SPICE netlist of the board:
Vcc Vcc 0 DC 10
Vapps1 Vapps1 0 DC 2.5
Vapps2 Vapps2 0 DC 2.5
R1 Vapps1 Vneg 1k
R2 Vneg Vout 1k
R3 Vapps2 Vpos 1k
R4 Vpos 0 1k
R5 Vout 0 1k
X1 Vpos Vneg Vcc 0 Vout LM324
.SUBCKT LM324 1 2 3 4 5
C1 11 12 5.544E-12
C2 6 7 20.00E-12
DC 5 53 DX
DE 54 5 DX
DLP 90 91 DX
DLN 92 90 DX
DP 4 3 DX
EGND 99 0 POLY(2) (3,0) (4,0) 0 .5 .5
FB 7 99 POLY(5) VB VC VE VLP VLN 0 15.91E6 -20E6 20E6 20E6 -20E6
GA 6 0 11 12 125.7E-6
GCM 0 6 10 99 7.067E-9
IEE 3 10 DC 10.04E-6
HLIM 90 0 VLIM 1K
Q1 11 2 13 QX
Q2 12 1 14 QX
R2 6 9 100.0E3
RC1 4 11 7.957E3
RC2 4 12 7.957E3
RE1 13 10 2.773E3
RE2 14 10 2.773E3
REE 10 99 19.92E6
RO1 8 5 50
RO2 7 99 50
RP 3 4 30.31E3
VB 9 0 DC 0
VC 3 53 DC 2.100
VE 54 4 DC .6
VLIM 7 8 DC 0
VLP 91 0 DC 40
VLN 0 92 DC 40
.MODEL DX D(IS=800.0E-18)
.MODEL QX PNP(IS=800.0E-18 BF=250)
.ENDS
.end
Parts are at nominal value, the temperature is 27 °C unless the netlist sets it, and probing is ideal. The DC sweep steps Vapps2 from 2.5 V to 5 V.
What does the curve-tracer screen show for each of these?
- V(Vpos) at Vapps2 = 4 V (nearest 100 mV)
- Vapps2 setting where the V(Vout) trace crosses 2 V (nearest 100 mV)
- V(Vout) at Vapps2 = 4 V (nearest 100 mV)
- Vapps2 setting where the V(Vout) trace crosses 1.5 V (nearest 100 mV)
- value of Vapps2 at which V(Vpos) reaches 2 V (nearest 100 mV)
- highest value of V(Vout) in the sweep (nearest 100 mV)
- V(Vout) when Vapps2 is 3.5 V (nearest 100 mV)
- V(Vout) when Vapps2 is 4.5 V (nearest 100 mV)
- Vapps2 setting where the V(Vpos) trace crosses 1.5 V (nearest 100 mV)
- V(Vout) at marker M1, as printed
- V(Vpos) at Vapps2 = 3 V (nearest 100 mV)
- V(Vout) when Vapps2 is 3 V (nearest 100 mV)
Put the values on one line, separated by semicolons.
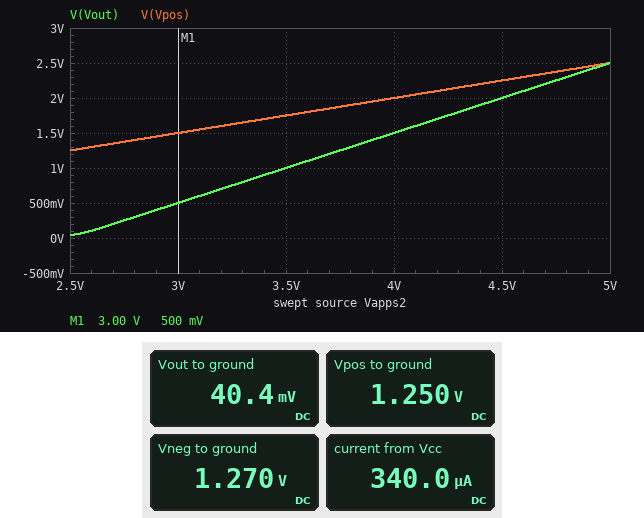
2.0 V; 4.5 V; 1.5 V; 4.0 V; 4.0 V; 2.5 V; 1.0 V; 2.0 V; 3.0 V; 500 mV; 1.5 V; 500 mV
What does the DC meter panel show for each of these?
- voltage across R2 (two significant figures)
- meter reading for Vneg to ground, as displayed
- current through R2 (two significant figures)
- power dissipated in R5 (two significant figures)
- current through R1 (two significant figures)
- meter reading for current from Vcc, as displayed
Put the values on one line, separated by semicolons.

1.2 V; 1.270 V; 1.2 mA; 1.6 µW; 1.2 mA; 340.0 µA
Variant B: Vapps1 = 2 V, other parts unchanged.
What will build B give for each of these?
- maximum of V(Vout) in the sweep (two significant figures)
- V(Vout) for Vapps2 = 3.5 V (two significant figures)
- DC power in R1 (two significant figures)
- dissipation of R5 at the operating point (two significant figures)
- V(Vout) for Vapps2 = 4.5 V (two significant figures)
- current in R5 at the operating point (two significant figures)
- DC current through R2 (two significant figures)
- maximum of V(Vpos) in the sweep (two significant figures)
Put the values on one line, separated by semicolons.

3.0 V; 1.5 V; 560 µW; 250 µW; 2.5 V; 500 µA; 750 µA; 2.5 V
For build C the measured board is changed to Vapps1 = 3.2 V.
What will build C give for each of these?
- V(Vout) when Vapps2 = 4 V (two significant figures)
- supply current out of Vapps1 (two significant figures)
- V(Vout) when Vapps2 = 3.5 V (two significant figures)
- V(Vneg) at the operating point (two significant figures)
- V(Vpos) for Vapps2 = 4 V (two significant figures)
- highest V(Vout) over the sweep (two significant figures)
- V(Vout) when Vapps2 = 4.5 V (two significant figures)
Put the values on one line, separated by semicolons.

800 mV; 1.6 mA; 300 mV; 1.6 V; 2.0 V; 1.8 V; 1.3 V
